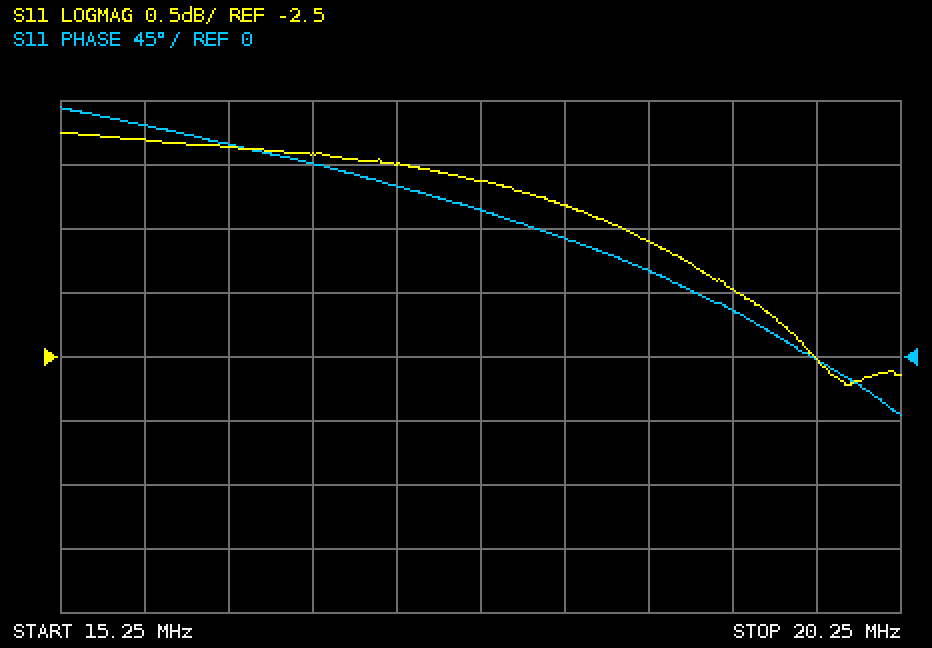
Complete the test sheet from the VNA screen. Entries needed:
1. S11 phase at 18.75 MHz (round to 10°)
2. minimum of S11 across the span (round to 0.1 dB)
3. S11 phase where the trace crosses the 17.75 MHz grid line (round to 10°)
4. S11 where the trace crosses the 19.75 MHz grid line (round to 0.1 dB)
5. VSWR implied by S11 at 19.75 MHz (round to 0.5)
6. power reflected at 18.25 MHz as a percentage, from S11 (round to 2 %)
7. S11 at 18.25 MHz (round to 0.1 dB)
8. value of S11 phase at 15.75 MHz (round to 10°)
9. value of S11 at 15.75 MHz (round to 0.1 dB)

60°
-2.7 dB
100°
-2.5 dB
7.0
74 %
-1.3 dB
160°
-0.8 dB
